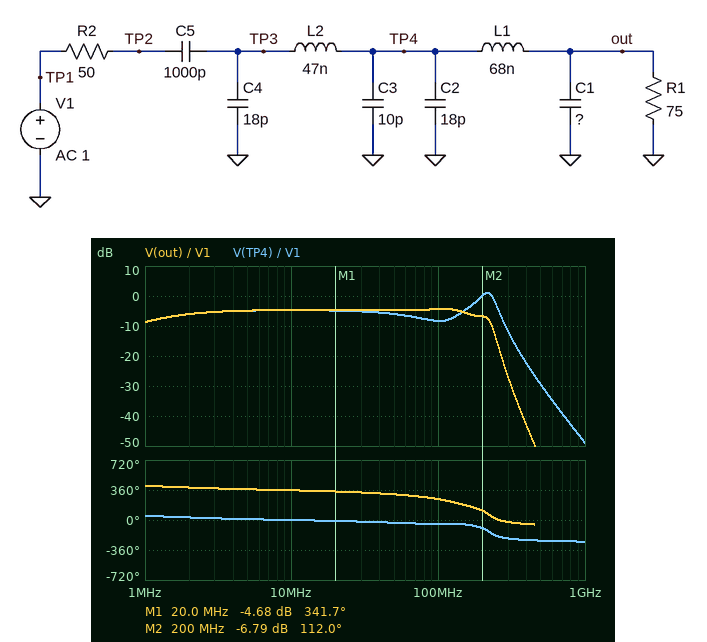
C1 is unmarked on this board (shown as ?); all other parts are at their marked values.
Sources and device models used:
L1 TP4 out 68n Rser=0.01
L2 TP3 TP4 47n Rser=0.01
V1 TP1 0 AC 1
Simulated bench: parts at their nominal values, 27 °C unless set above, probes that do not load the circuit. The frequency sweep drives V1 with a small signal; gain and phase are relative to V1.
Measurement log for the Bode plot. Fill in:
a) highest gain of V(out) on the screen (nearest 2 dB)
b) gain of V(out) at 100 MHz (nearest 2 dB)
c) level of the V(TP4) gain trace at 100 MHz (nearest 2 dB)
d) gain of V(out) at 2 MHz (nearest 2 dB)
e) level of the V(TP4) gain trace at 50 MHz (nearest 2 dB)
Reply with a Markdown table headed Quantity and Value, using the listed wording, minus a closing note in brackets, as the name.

| Quantity | Value |
|---|---|
| highest gain of V(out) on the screen | -4 dB |
| gain of V(out) at 100 MHz | -4 dB |
| level of the V(TP4) gain trace at 100 MHz | -8 dB |
| gain of V(out) at 2 MHz | -6 dB |
| level of the V(TP4) gain trace at 50 MHz | -6 dB |
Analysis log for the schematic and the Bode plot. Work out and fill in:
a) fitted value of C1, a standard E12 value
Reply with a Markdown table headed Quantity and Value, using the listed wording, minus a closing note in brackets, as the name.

| Quantity | Value |
|---|---|
| fitted value of C1, a standard E12 value | 27 pF |
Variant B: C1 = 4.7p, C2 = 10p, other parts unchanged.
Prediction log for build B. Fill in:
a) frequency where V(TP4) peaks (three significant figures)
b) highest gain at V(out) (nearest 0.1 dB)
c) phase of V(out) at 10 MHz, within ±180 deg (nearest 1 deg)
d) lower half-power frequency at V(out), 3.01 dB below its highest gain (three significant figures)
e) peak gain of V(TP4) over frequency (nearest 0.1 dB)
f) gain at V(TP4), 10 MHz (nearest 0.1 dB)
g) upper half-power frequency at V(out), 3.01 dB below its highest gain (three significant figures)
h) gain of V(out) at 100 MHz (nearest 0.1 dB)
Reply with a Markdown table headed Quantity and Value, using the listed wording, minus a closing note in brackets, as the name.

| Quantity | Value |
|---|---|
| frequency where V(TP4) peaks | 239 MHz |
| highest gain at V(out) | -4.3 dB |
| phase of V(out) at 10 MHz, within ±180 deg | -1 deg |
| lower half-power frequency at V(out), 3.01 dB below its highest gain | 1.33 MHz |
| peak gain of V(TP4) over frequency | -1.6 dB |
| gain at V(TP4), 10 MHz | -4.6 dB |
| upper half-power frequency at V(out), 3.01 dB below its highest gain | 272 MHz |
| gain of V(out) at 100 MHz | -4.9 dB |
